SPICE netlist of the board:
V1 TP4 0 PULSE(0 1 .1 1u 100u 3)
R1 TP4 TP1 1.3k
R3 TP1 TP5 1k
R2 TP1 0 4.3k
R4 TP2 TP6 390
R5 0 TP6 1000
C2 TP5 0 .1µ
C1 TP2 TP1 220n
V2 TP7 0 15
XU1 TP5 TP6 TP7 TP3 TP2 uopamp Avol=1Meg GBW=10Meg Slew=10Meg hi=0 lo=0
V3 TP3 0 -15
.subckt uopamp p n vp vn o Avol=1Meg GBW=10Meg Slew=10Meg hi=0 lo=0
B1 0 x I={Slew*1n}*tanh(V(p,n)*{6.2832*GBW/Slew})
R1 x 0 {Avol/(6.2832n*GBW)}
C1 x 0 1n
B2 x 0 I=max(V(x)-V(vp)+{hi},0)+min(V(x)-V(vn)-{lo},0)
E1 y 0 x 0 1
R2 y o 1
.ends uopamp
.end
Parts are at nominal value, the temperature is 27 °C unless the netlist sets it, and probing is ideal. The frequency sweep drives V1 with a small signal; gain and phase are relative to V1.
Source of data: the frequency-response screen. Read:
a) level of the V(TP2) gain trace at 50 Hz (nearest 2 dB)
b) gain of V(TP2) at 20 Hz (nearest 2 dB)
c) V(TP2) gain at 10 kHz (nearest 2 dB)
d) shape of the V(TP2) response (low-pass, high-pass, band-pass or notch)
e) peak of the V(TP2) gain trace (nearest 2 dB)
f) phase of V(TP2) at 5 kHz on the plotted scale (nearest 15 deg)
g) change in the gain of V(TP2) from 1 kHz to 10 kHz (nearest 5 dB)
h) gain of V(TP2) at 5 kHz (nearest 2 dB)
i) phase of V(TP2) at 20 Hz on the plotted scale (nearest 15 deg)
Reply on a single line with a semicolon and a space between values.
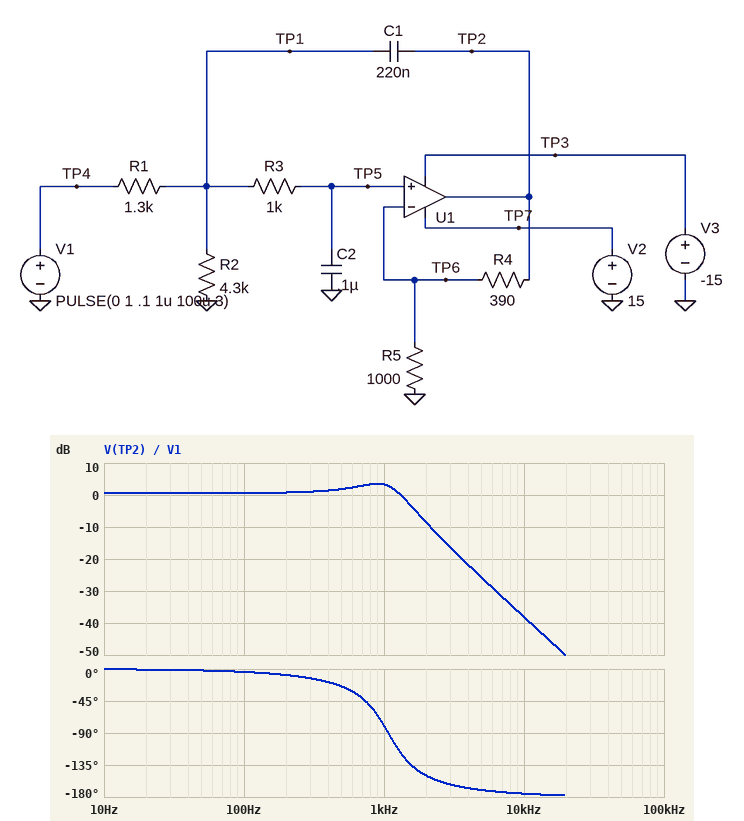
0 dB; 0 dB; -38 dB; low-pass; 4 dB; -165 deg; -40 dB; -26 dB; 0 deg
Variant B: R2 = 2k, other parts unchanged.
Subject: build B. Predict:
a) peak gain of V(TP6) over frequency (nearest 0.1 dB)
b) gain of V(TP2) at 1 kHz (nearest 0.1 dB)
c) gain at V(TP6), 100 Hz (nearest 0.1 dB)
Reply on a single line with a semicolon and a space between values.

-2.0 dB; 0.8 dB; -4.3 dB
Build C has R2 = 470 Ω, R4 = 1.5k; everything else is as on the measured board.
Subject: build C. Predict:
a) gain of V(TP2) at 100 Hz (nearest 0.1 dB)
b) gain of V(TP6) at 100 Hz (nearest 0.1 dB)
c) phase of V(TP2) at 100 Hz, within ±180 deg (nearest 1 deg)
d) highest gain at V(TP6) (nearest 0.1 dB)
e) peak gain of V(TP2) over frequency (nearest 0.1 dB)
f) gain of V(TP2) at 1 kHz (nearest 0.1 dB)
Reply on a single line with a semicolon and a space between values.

-3.5 dB; -11.5 dB; -1 deg; 1.1 dB; 9.0 dB; -0.6 dB
